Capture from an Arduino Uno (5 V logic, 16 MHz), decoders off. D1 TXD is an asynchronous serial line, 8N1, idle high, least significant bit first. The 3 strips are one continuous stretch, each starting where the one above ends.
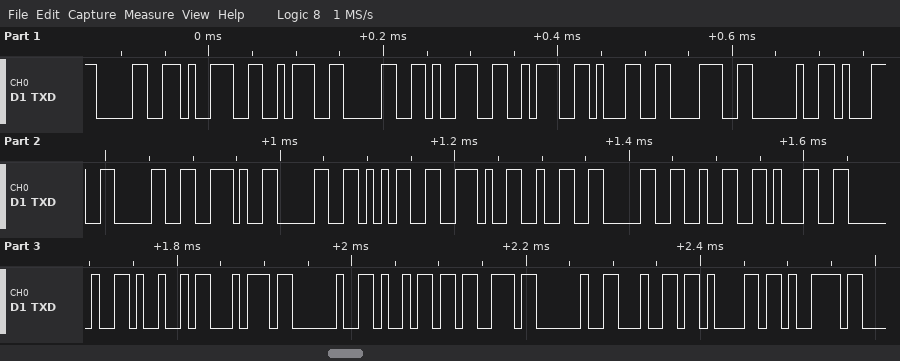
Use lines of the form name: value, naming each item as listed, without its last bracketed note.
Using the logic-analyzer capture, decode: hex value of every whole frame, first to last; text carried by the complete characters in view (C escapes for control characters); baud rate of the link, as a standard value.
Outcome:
hex value of every whole frame, first to last: 0x30 0x39 0x3A 0x30 0x39 0x3A 0x31 0x38 0x20 0x31 0x30 0x2E 0x30 0x35 0x2E 0x32 0x30 0x32 0x31 0x20 0x49 0x74 0x20 0x69 0x73 0x20 0x64 0x61 0x79
text carried by the complete characters in view: "09:09:18 10.05.2021 It is day"
baud rate of the link, as a standard value: 115200 baud
